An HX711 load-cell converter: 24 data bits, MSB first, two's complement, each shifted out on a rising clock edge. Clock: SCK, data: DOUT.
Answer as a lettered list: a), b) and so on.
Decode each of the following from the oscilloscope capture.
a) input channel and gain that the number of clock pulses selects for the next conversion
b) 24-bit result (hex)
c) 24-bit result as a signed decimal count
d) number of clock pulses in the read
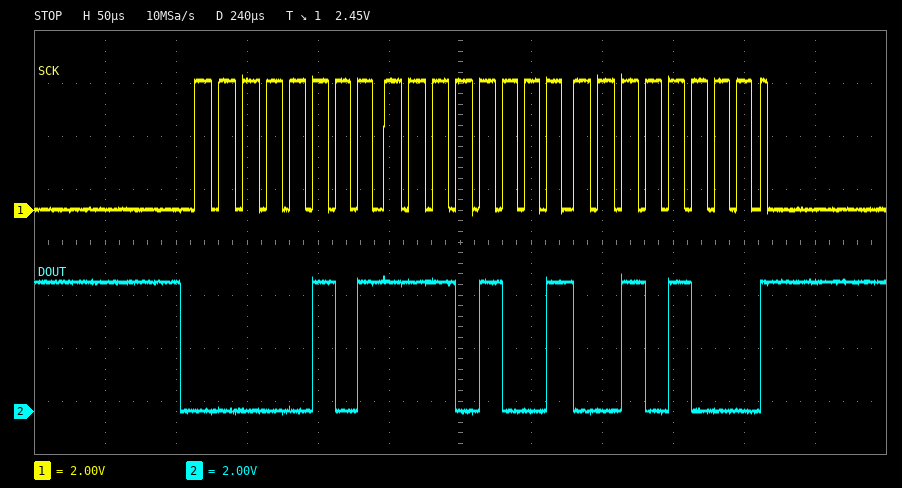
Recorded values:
a) channel A, gain 128
b) 0x05E928
c) 387368
d) 25
